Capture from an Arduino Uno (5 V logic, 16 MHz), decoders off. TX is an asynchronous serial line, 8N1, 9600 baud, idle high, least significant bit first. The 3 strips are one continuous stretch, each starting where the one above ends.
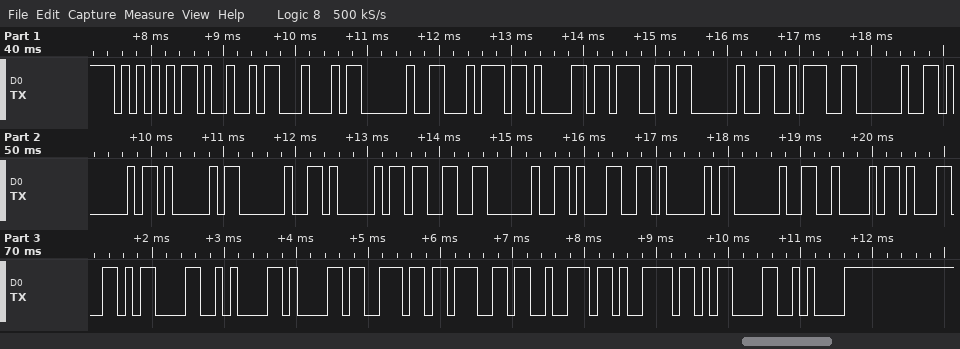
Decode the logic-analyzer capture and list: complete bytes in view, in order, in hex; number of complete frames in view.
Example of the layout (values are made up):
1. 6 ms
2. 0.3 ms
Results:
1. 55 49 44 20 74 61 67 20 3A 20 41 41 20 41 33 20 31 41 20 42 31 0D 0A 61 6E 67 72 79 0D 0A
2. 30
